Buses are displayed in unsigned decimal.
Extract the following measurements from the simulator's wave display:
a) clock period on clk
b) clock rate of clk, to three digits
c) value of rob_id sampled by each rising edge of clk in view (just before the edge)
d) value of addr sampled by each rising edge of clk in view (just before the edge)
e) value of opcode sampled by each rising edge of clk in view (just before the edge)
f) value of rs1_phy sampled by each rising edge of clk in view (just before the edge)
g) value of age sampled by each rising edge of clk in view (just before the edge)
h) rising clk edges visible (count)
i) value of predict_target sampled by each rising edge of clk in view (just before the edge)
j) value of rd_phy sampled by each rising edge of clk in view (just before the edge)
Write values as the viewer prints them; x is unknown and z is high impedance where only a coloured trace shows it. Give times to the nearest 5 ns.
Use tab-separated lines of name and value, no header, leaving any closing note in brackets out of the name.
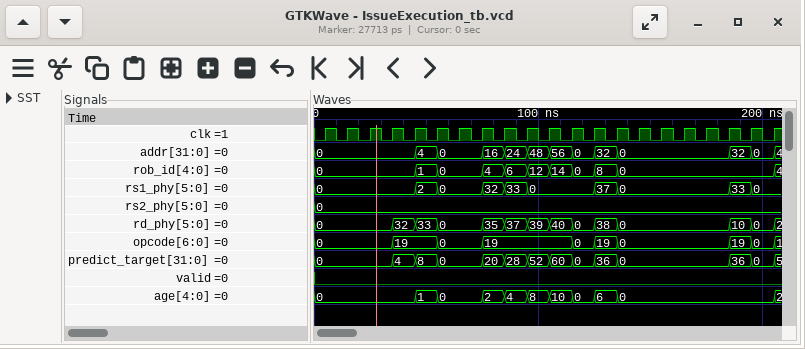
clock period on clk	10 ns
clock rate of clk, to three digits	100 MHz
value of rob_id sampled by each rising edge of clk in view	0, 0, 0, 0, 0, 1, 0, 0, 4, 6, 12, 14, 0, 8, 0, 0, 0, 0, 0, 0, 0
value of addr sampled by each rising edge of clk in view	0, 0, 0, 0, 0, 4, 0, 0, 16, 24, 48, 56, 0, 32, 0, 0, 0, 0, 0, 32, 0
value of opcode sampled by each rising edge of clk in view	0, 0, 0, 0, 19, 19, 0, 0, 19, 19, 19, 19, 0, 19, 0, 0, 0, 0, 0, 19, 0
value of rs1_phy sampled by each rising edge of clk in view	0, 0, 0, 0, 0, 2, 0, 0, 32, 33, 0, 0, 0, 37, 0, 0, 0, 0, 0, 33, 0
value of age sampled by each rising edge of clk in view	0, 0, 0, 0, 0, 1, 0, 0, 2, 4, 8, 10, 0, 6, 0, 0, 0, 0, 0, 0, 0
rising clk edges visible	21
value of predict_target sampled by each rising edge of clk in view	0, 0, 0, 0, 4, 8, 0, 0, 20, 28, 52, 60, 0, 36, 0, 0, 0, 0, 0, 36, 0
value of rd_phy sampled by each rising edge of clk in view	0, 0, 0, 0, 32, 33, 0, 0, 35, 37, 39, 40, 0, 38, 0, 0, 0, 0, 0, 10, 0
